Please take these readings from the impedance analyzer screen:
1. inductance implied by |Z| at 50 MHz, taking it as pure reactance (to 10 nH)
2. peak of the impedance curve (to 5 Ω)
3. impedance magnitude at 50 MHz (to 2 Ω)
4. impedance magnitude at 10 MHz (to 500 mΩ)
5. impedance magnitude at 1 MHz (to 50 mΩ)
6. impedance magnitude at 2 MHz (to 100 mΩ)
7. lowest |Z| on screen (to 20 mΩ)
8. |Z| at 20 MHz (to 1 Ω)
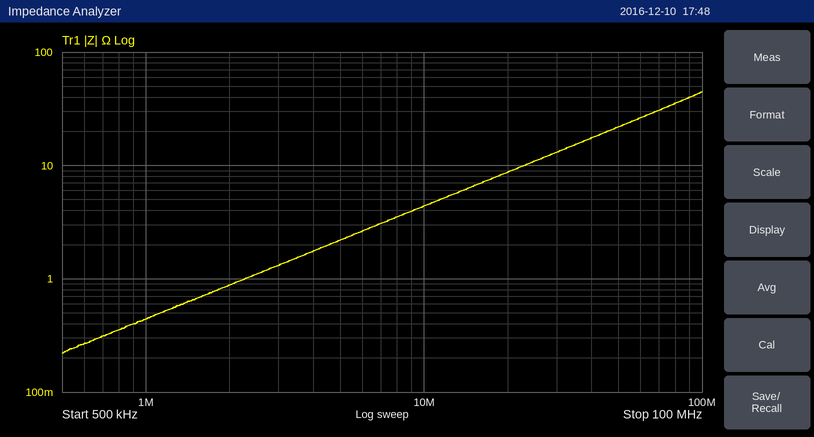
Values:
70 nH
45 Ω
22 Ω
4.5 Ω
450 mΩ
900 mΩ
220 mΩ
9 Ω
